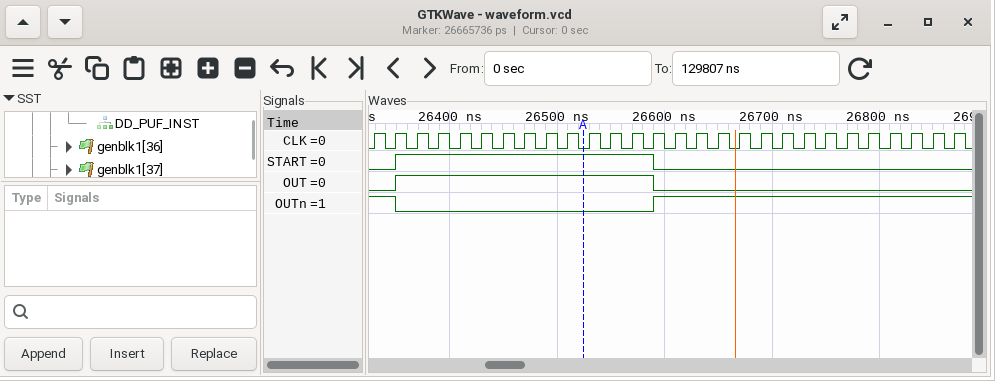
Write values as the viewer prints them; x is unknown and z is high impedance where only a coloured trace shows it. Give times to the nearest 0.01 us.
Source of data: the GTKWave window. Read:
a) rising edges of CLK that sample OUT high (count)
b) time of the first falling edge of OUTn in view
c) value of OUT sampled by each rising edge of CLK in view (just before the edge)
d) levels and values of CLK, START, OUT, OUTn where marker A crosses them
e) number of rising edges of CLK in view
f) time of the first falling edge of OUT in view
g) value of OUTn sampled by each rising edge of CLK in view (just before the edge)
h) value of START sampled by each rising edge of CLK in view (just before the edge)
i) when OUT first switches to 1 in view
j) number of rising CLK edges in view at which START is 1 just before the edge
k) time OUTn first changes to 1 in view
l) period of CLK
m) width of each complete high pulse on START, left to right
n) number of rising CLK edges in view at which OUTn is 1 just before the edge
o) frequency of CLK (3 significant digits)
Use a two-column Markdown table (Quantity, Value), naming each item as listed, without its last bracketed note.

| Quantity | Value |
|---|---|
| rising edges of CLK that sample OUT high | 12 |
| time of the first falling edge of OUTn in view | 26.35 us |
| value of OUT sampled by each rising edge of CLK in view | 0 0 1 1 1 1 1 1 1 1 1 1 1 1 0 0 0 0 0 0 0 0 0 0 0 0 0 0 |
| levels and values of CLK, START, OUT, OUTn where marker A crosses them | CLK=0, START=1, OUT=1, OUTn=0 |
| number of rising edges of CLK in view | 28 |
| time of the first falling edge of OUT in view | 26.59 us |
| value of OUTn sampled by each rising edge of CLK in view | 1 1 0 0 0 0 0 0 0 0 0 0 0 0 1 1 1 1 1 1 1 1 1 1 1 1 1 1 |
| value of START sampled by each rising edge of CLK in view | 0 0 1 1 1 1 1 1 1 1 1 1 1 1 0 0 0 0 0 0 0 0 0 0 0 0 0 0 |
| when OUT first switches to 1 in view | 26.35 us |
| number of rising CLK edges in view at which START is 1 just before the edge | 12 |
| time OUTn first changes to 1 in view | 26.59 us |
| period of CLK | 0.02 us |
| width of each complete high pulse on START, left to right | 0.24 us |
| number of rising CLK edges in view at which OUTn is 1 just before the edge | 16 |
| frequency of CLK | 50.0 MHz |
